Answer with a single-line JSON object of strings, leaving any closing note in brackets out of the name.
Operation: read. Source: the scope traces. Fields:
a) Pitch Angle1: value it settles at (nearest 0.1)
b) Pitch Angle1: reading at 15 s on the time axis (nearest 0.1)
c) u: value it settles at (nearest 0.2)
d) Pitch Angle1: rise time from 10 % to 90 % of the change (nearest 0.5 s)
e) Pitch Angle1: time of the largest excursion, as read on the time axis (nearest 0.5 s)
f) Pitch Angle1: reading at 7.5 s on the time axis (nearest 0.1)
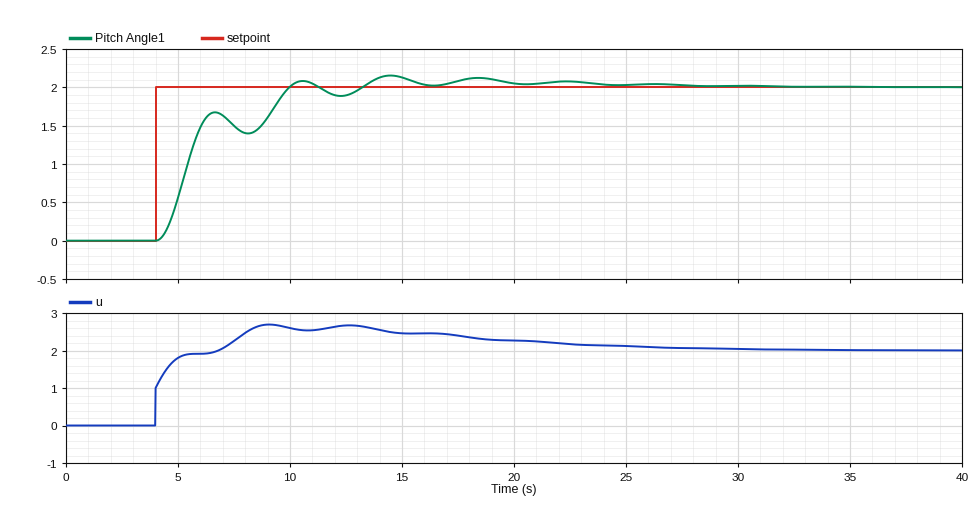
{"Pitch Angle1: value it settles at": "2.0", "Pitch Angle1: reading at 15 s on the time axis": "2.1", "u: value it settles at": "2.0", "Pitch Angle1: rise time from 10 % to 90 % of the change": "5.0 s", "Pitch Angle1: time of the largest excursion, as read on the time axis": "14.5 s", "Pitch Angle1: reading at 7.5 s on the time axis": "1.5"}
